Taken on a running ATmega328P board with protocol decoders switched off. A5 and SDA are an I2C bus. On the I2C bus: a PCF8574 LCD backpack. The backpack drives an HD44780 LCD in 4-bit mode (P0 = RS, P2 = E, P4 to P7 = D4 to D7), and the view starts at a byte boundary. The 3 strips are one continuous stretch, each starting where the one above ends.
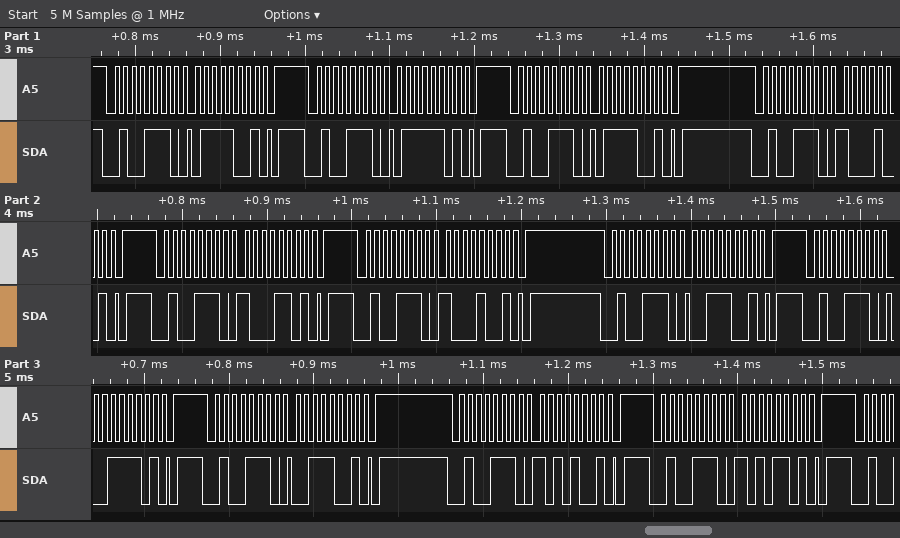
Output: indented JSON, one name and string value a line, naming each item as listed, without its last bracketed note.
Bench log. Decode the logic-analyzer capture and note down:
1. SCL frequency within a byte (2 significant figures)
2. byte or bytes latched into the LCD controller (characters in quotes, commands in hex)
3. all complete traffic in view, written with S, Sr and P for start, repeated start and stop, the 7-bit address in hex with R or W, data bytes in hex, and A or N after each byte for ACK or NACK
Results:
{
  "SCL frequency within a byte": "100 kHz",
  "byte or bytes latched into the LCD controller": "'x'",
  "all complete traffic in view, written with S, Sr and P for start, repeated start and stop, the 7-bit address in hex with R or W, data bytes in hex, and A or N after each byte for ACK or NACK": "S 27W A 79 A P S 27W A 7D A P S 27W A 79 A P S 27W A 89 A P S 27W A 8D A P S 27W A 89 A P S 27W A 39 A P S 27W A 3D A P S 27W A 39 A P S 27W A A9 A P S 27W A AD A P"
}
